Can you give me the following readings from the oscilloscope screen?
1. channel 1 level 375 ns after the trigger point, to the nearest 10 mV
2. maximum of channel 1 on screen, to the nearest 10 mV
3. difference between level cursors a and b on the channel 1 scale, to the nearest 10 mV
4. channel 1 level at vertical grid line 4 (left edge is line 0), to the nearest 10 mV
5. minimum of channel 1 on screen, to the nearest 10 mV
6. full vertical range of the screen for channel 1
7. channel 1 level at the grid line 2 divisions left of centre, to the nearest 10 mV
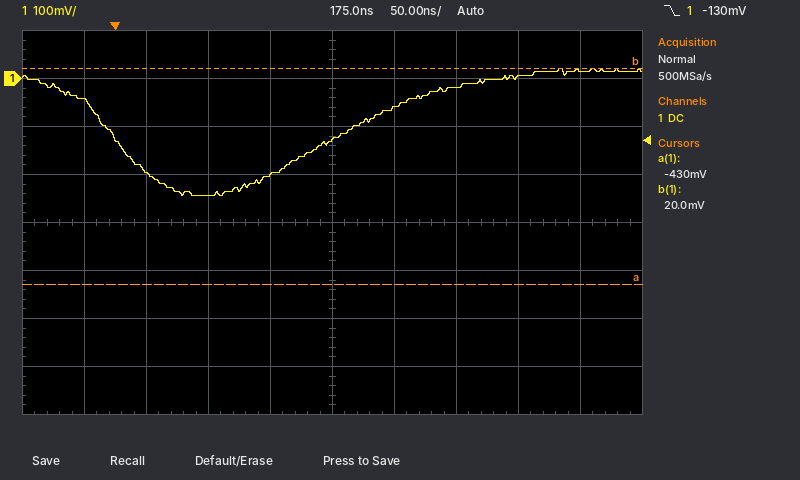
20 mV
20 mV
450 mV
-200 mV
-240 mV
800 mV
-240 mV
